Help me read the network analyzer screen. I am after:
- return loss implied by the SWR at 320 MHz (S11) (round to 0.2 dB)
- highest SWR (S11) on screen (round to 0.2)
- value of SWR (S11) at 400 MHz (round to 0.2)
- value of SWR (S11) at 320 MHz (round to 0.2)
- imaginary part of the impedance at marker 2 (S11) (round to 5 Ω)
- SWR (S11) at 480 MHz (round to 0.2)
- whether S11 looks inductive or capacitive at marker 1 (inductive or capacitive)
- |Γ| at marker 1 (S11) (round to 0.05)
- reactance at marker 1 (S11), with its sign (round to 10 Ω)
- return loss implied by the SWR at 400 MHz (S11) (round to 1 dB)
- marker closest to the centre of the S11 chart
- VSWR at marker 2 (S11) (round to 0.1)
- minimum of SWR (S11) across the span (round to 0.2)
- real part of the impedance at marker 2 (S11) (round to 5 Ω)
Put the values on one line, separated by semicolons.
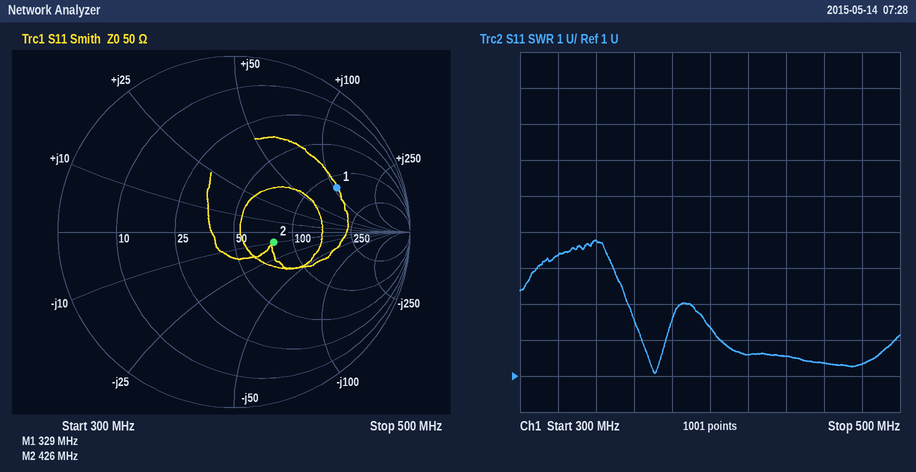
4.0 dB; 4.8; 2.4; 4.4; -10 Ω; 1.4; inductive; 0.65; +110 Ω; 8 dB; marker 2; 1.6; 1.0; 80 Ω
